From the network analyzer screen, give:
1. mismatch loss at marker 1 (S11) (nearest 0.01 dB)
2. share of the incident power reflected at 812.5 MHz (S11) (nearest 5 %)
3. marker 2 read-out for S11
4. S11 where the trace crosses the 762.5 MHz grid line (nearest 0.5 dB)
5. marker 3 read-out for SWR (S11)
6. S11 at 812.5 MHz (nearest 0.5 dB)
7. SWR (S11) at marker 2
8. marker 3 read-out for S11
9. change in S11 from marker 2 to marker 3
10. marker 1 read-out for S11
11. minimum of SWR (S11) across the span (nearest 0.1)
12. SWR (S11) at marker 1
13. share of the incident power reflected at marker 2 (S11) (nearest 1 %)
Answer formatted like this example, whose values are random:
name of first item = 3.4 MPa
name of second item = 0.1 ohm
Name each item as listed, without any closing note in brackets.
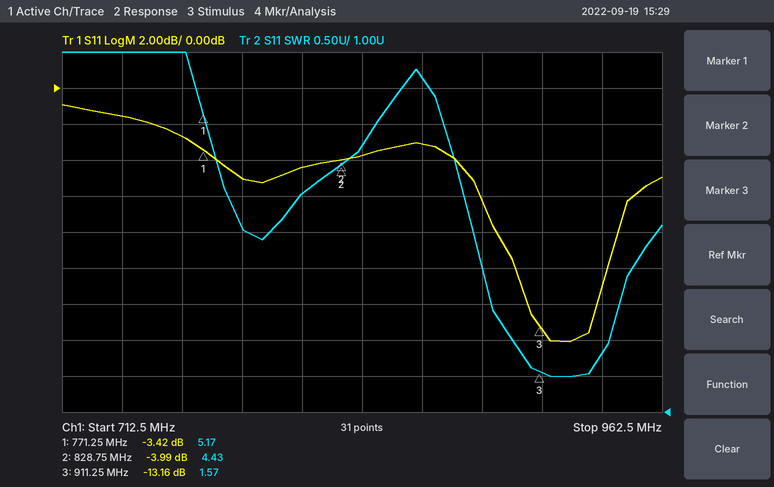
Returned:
mismatch loss at marker 1 (S11) = 2.64 dB
share of the incident power reflected at 812.5 MHz (S11) = 35 %
marker 2 read-out for S11 = -3.99 dB
S11 where the trace crosses the 762.5 MHz grid line = -2.5 dB
marker 3 read-out for SWR = 1.57
S11 at 812.5 MHz = -4.5 dB
SWR (S11) at marker 2 = 4.43
marker 3 read-out for S11 = -13.16 dB
change in S11 from marker 2 to marker 3 = -9.17 dB
marker 1 read-out for S11 = -3.42 dB
minimum of SWR (S11) across the span = 1.5
SWR (S11) at marker 1 = 5.17
share of the incident power reflected at marker 2 (S11) = 40 %
